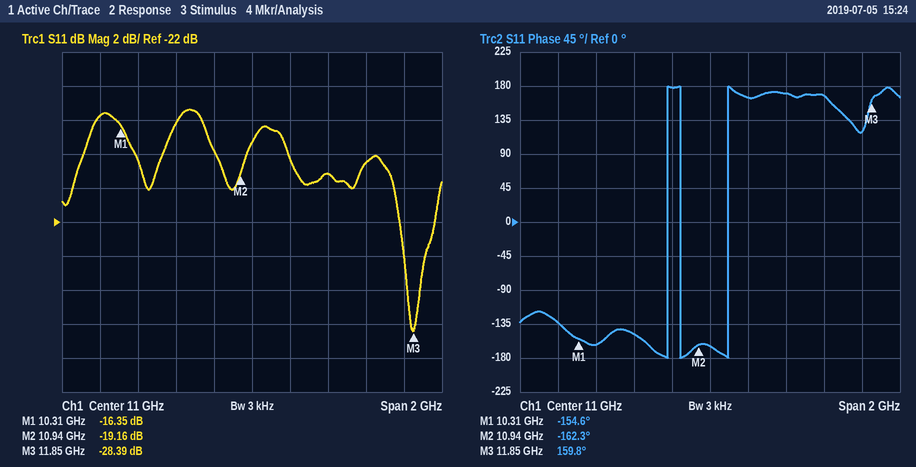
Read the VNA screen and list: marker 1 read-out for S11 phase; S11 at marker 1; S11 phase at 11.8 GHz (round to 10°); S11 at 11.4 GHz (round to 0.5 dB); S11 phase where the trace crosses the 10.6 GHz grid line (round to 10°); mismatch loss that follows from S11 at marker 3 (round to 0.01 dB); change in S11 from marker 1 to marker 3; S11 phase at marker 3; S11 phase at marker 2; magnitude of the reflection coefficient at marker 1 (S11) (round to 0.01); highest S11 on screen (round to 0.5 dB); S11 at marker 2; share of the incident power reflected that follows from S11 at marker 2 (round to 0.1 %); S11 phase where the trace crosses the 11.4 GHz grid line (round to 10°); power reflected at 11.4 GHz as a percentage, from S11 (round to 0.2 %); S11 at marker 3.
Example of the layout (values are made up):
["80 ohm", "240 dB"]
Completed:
["-154.6°", "-16.35 dB", "120°", "-19.0 dB", "-150°", "0.01 dB", "-12.04 dB", "159.8°", "-162.3°", "0.15", "-15.5 dB", "-19.16 dB", "1.2 %", "170°", "1.2 %", "-28.39 dB"]
